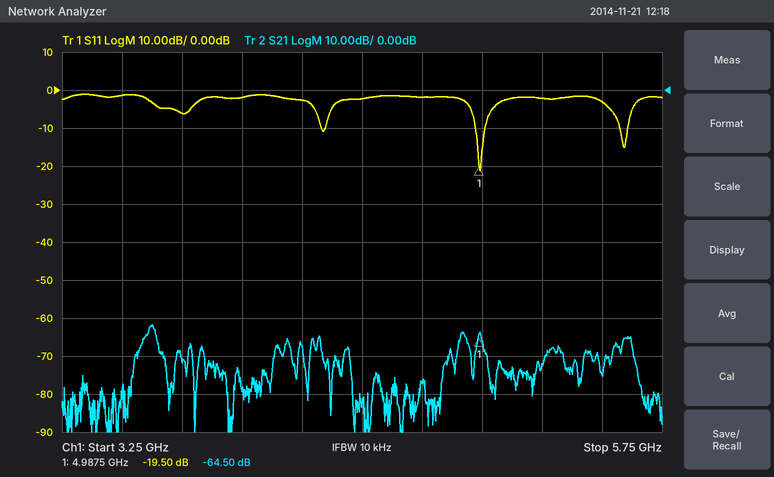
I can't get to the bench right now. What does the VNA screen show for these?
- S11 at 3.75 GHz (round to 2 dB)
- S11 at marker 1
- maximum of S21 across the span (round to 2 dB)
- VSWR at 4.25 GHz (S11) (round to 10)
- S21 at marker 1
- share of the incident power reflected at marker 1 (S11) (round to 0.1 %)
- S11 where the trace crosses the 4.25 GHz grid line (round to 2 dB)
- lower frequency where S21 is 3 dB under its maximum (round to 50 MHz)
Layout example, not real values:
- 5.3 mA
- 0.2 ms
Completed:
- -6 dB
- -19.50 dB
- -62 dB
- 10
- -64.50 dB
- 1.1 %
- -2 dB
- 3.60 GHz
